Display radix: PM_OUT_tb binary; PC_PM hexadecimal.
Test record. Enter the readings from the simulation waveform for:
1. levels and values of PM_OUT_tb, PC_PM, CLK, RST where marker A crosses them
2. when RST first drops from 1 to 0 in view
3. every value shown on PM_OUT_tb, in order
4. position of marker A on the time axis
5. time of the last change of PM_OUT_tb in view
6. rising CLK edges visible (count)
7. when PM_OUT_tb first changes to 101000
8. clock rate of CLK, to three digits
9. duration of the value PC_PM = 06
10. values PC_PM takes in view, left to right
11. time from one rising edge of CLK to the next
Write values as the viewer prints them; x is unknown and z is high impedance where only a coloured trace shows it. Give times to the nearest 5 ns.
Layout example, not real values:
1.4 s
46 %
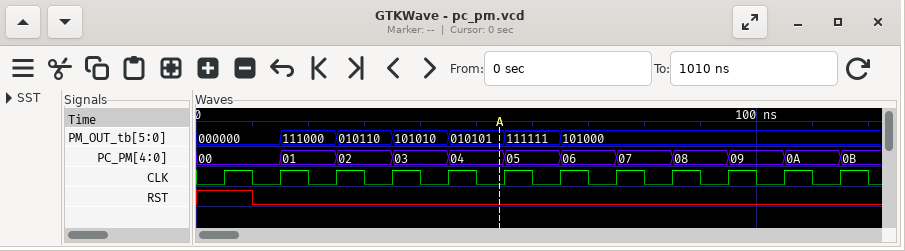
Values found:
PM_OUT_tb=010101, PC_PM=04, CLK=0, RST=0
10 ns
000000, 111000, 010110, 101010, 010101, 111111, 101000
55 ns
65 ns
12
65 ns
100 MHz
10 ns
00, 01, 02, 03, 04, 05, 06, 07, 08, 09, 0A, 0B
10 ns
